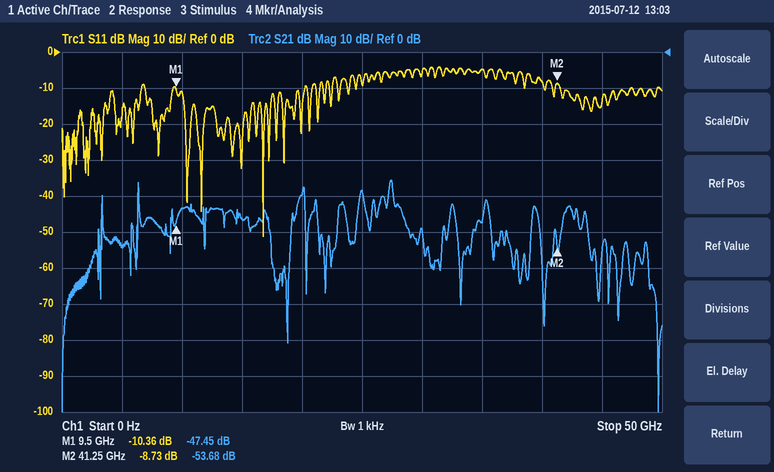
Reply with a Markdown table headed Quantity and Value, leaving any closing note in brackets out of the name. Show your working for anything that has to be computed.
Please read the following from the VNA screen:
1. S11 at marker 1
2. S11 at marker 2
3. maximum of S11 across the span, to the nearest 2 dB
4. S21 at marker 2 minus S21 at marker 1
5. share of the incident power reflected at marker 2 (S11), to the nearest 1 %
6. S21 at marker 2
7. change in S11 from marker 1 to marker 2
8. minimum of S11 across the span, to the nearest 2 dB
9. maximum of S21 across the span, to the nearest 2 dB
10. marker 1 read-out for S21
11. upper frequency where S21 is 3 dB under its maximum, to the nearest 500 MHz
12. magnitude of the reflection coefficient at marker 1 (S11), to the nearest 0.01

| Quantity | Value |
|---|---|
| S11 at marker 1 | -10.36 dB |
| S11 at marker 2 | -8.73 dB |
| maximum of S11 across the span, to the nearest 2 dB | -4 dB |
| S21 at marker 2 minus S21 at marker 1 | -53.68 − (-47.45) = -6.23 dB |
| share of the incident power reflected at marker 2 (S11), to the nearest 1 % | 10^(-8.73/10) ≈ 13 % |
| S21 at marker 2 | -53.68 dB |
| change in S11 from marker 1 to marker 2 | -8.73 − (-10.36) = 1.63 dB |
| minimum of S11 across the span, to the nearest 2 dB | -52 dB |
| maximum of S21 across the span, to the nearest 2 dB | -36 dB |
| marker 1 read-out for S21 | -47.45 dB |
| upper frequency where S21 is 3 dB under its maximum, to the nearest 500 MHz | 27.5 GHz |
| magnitude of the reflection coefficient at marker 1 (S11), to the nearest 0.01 | 10^(-10.36/20) ≈ 0.30 |
